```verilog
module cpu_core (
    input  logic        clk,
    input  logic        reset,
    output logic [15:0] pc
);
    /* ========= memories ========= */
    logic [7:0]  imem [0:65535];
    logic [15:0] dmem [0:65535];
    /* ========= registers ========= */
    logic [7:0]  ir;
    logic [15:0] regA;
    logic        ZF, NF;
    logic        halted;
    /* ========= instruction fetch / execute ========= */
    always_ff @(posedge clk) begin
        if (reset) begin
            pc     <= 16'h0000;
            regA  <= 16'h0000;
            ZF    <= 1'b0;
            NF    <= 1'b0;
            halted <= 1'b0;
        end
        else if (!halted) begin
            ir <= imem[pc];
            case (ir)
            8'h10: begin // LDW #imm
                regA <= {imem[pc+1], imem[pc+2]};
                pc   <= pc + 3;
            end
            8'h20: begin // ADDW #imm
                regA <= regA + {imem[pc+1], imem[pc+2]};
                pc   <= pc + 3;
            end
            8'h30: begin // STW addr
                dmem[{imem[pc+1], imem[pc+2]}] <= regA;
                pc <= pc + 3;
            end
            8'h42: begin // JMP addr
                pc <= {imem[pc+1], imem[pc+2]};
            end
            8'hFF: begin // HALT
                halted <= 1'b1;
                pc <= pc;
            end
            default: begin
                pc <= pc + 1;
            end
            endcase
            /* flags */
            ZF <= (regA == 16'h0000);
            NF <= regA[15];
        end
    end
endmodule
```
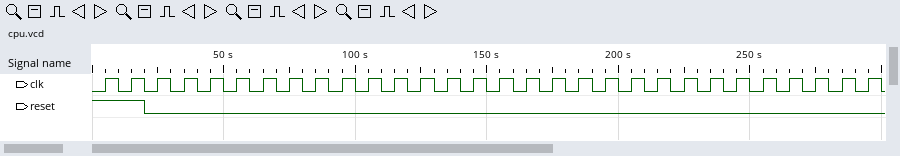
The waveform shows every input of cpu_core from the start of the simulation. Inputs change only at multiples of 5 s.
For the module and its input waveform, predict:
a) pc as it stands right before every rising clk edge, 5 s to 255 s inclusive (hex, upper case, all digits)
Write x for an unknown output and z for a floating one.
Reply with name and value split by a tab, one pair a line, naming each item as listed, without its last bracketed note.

pc as it stands right before every rising clk edge, 5 s to 255 s inclusive	x, 0000, 0000, 0001, 0002, 0003, 0004, 0005, 0006, 0007, 0008, 0009, 000A, 000B, 000C, 000D, 000E, 000F, 0010, 0011, 0012, 0013, 0014, 0015, 0016, 0017
